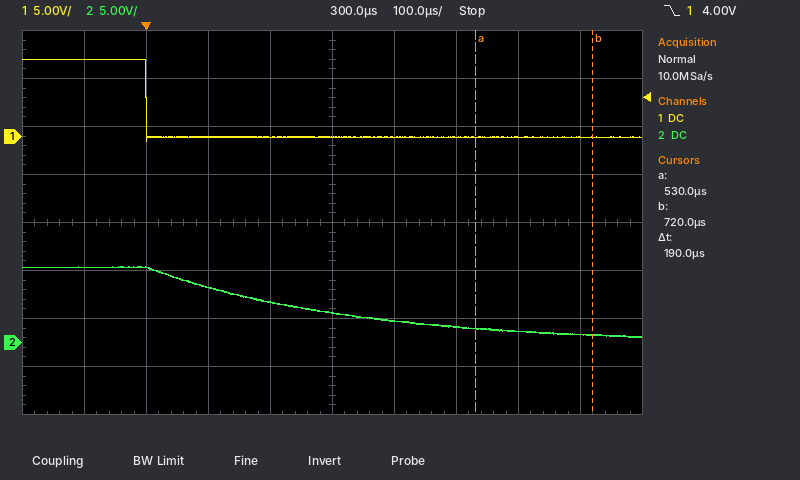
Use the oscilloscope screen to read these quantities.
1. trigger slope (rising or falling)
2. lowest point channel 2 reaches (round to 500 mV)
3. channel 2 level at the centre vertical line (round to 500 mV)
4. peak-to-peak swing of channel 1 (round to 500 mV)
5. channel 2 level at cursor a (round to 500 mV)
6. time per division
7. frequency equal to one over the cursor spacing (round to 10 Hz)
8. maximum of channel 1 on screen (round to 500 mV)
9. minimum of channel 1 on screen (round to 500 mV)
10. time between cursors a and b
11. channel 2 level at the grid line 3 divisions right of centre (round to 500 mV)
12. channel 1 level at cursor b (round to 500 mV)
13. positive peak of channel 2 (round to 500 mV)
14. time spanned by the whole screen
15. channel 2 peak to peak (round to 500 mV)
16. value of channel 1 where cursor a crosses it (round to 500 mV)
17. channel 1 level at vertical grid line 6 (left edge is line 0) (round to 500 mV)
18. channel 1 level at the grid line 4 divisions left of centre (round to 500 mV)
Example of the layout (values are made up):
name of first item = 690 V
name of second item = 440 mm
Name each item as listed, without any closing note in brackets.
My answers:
trigger slope = falling
lowest point channel 2 reaches = 500 mV
channel 2 level at the centre vertical line = 3.0 V
peak-to-peak swing of channel 1 = 8.5 V
channel 2 level at cursor a = 1.5 V
time per division = 100 µs
frequency equal to one over the cursor spacing = 5.26 kHz
maximum of channel 1 on screen = 8.0 V
minimum of channel 1 on screen = -500 mV
time between cursors a and b = 190 µs
channel 2 level at the grid line 3 divisions right of centre = 1.0 V
channel 1 level at cursor b = 0.0 V
positive peak of channel 2 = 8.0 V
time spanned by the whole screen = 1 ms
channel 2 peak to peak = 7.5 V
value of channel 1 where cursor a crosses it = 0.0 V
channel 1 level at vertical grid line 6 (left edge is line 0) = 0.0 V
channel 1 level at the grid line 4 divisions left of centre = 8.0 V
